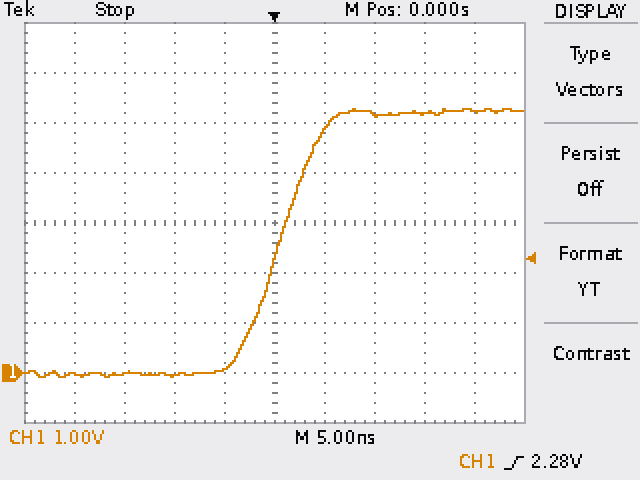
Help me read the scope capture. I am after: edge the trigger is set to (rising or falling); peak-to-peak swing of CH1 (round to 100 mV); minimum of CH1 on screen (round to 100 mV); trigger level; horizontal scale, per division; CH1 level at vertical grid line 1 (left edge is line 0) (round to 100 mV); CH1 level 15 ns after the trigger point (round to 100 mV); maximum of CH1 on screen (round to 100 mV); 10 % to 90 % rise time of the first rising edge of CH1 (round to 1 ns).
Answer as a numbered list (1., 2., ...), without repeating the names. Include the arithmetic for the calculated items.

1. rising
2. 5.3 V − (-100 mV) = 5.4 V
3. -100 mV
4. 2.28 V
5. 5 ns
6. 0.0 V
7. 5.2 V
8. 5.3 V
9. 8 ns
